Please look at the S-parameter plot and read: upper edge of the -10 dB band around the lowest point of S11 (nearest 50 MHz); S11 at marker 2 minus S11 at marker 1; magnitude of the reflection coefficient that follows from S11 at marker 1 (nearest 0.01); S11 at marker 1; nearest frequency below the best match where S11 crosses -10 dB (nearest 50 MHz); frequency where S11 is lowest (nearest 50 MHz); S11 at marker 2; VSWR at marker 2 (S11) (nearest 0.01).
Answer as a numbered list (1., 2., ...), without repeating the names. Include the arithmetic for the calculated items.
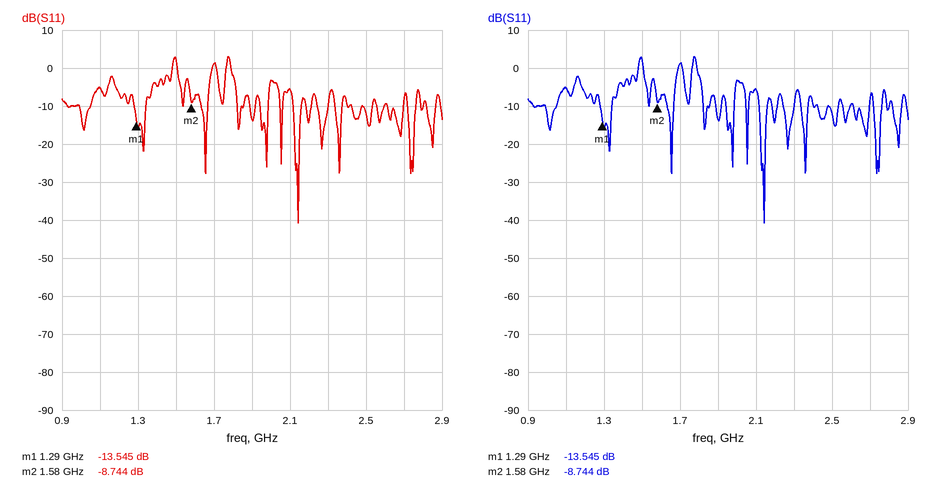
1. 2.15 GHz
2. -8.744 − (-13.545) = 4.801 dB
3. 10^(-13.545/20) ≈ 0.21
4. -13.545 dB
5. 2.10 GHz
6. 2.15 GHz
7. -8.744 dB
8. (1 + 0.3654)/(1 − 0.3654) ≈ 2.15
